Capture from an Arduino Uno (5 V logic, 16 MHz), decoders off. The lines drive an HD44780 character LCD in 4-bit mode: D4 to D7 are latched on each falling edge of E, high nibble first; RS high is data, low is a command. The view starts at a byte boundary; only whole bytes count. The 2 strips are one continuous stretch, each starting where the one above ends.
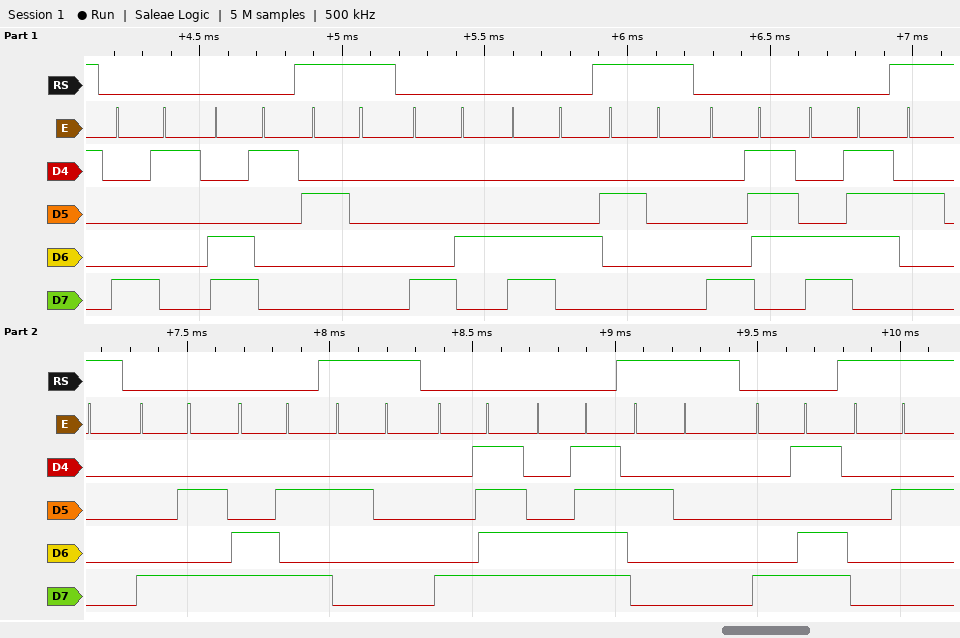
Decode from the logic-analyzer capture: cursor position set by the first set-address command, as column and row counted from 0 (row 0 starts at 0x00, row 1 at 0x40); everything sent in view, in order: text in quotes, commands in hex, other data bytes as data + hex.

column 1, row 0
0x81 0xC1 " " 0x84 0xC4 " " 0x87 0xC7 " " 0x8A 0xCA " " 0x8F 0xCF " " 0x8D data 02
